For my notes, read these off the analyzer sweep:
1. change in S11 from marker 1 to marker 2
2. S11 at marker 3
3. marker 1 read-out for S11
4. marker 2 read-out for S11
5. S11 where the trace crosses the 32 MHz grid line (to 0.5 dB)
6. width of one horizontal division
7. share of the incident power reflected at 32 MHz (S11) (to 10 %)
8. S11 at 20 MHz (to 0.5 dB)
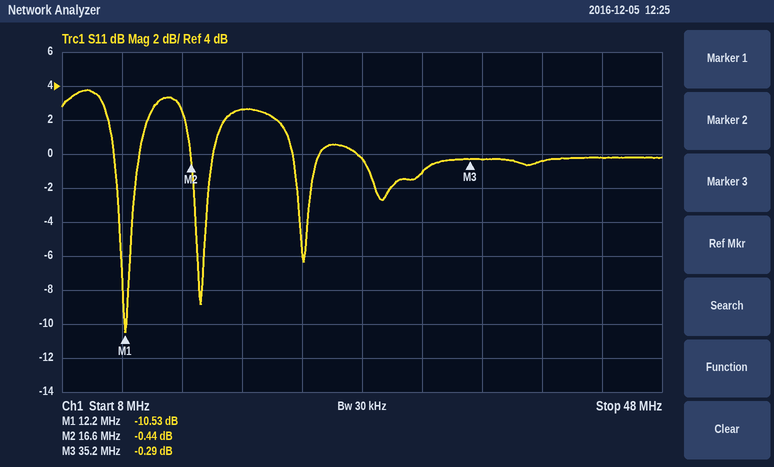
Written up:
10.09 dB
-0.29 dB
-10.53 dB
-0.44 dB
-1.0 dB
4 MHz
80 %
2.5 dB
